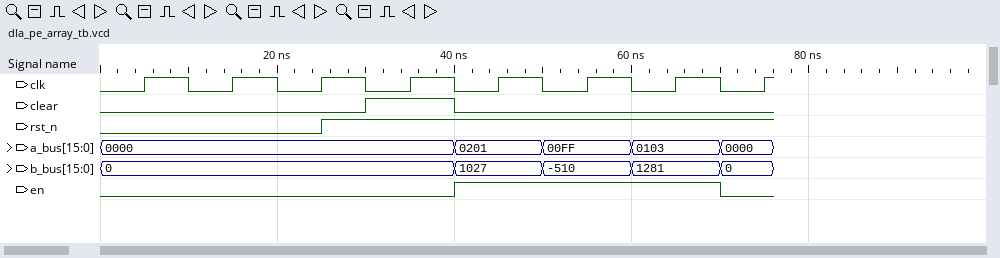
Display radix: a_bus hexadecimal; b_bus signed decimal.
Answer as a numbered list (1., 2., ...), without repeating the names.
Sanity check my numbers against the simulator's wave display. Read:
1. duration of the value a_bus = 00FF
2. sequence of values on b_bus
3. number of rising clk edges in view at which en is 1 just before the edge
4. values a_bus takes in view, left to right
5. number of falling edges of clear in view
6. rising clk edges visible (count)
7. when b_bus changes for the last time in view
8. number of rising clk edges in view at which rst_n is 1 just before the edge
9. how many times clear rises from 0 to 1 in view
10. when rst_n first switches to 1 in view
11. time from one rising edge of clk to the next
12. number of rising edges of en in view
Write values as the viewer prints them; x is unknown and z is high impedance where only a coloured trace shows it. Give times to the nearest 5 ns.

1. 10 ns
2. 0, 1027, -510, 1281, 0
3. 3
4. 0000, 0201, 00FF, 0103, 0000
5. 1
6. 8
7. 70 ns
8. 5
9. 1
10. 25 ns
11. 10 ns
12. 1
